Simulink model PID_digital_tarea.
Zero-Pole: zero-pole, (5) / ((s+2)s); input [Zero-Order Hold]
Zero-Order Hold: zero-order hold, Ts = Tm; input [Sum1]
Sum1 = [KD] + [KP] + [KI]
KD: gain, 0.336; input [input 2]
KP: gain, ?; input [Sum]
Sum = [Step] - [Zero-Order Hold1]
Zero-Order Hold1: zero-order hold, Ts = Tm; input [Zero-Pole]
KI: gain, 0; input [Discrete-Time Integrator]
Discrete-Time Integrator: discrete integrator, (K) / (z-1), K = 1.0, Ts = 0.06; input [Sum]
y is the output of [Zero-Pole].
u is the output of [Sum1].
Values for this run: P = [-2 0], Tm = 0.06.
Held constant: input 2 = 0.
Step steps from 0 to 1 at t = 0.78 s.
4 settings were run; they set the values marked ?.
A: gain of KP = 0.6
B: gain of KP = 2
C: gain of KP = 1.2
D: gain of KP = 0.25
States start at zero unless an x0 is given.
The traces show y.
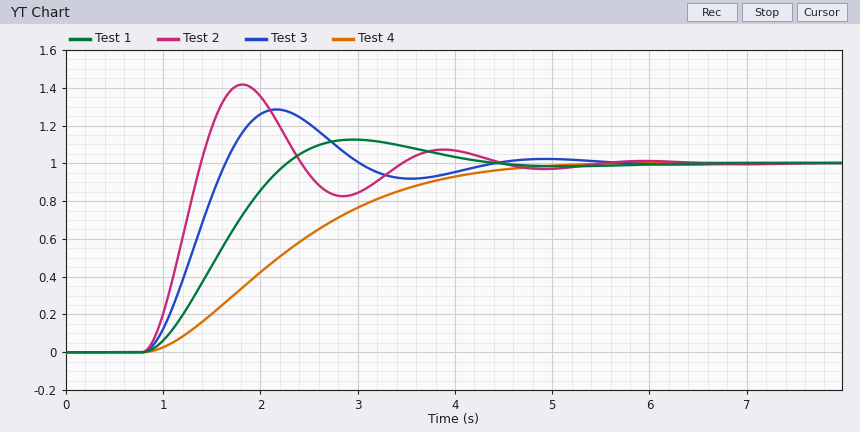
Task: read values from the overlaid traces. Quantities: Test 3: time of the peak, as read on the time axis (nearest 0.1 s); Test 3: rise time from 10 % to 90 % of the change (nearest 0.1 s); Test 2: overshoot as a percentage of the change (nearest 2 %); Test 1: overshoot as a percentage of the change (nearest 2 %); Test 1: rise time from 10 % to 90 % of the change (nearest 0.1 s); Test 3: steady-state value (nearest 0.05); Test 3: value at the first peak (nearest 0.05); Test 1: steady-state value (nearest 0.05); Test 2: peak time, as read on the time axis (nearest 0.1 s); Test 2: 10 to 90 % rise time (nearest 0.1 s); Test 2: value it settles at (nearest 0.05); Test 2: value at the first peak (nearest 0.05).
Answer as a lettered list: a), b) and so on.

a) 2.2 s
b) 0.6 s
c) 42 %
d) 12 %
e) 1.0 s
f) 1.00
g) 1.30
h) 1.00
i) 1.8 s
j) 0.4 s
k) 1.00
l) 1.40
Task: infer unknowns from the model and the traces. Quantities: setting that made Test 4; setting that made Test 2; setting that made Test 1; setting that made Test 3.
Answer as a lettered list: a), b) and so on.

a) D
b) B
c) A
d) C
